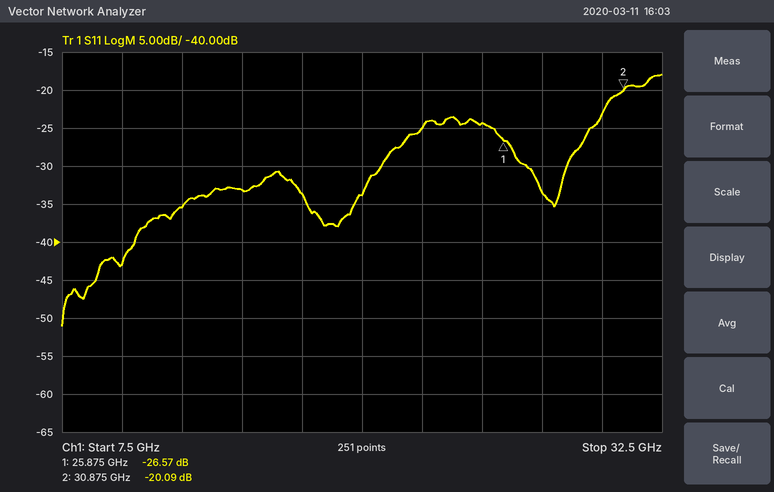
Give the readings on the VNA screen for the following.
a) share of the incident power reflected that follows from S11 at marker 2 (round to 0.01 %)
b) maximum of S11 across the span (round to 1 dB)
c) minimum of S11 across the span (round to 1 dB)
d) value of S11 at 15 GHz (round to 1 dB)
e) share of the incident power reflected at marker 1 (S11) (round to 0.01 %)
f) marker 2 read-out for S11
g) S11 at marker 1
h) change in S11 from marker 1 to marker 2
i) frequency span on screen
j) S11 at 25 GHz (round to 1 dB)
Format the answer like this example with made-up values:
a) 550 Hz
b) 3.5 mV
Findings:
a) 0.98 %
b) -18 dB
c) -51 dB
d) -33 dB
e) 0.22 %
f) -20.09 dB
g) -26.57 dB
h) 6.48 dB
i) 25 GHz
j) -24 dB
